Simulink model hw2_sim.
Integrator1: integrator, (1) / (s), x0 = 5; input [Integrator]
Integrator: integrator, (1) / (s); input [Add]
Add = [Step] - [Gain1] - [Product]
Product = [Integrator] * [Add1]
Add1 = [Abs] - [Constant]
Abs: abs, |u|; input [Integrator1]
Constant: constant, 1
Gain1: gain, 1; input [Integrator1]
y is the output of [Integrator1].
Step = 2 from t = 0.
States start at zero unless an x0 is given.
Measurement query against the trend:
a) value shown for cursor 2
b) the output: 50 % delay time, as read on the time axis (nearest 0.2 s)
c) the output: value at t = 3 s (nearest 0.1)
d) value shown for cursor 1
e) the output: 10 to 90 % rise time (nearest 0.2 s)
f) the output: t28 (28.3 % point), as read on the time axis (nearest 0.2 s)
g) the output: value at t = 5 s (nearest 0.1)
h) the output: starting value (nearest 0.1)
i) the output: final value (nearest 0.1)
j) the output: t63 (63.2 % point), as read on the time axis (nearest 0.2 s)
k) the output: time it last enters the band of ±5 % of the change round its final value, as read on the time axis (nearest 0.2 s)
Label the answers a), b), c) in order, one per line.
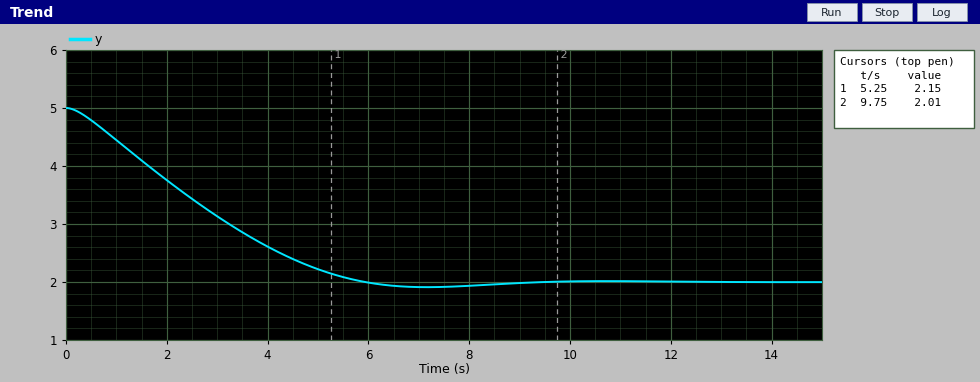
a) 2.01
b) 2.4 s
c) 3.1
d) 2.15
e) 4.2 s
f) 1.4 s
g) 2.2
h) 5.0
i) 2.0
j) 3.0 s
k) 5.2 s
